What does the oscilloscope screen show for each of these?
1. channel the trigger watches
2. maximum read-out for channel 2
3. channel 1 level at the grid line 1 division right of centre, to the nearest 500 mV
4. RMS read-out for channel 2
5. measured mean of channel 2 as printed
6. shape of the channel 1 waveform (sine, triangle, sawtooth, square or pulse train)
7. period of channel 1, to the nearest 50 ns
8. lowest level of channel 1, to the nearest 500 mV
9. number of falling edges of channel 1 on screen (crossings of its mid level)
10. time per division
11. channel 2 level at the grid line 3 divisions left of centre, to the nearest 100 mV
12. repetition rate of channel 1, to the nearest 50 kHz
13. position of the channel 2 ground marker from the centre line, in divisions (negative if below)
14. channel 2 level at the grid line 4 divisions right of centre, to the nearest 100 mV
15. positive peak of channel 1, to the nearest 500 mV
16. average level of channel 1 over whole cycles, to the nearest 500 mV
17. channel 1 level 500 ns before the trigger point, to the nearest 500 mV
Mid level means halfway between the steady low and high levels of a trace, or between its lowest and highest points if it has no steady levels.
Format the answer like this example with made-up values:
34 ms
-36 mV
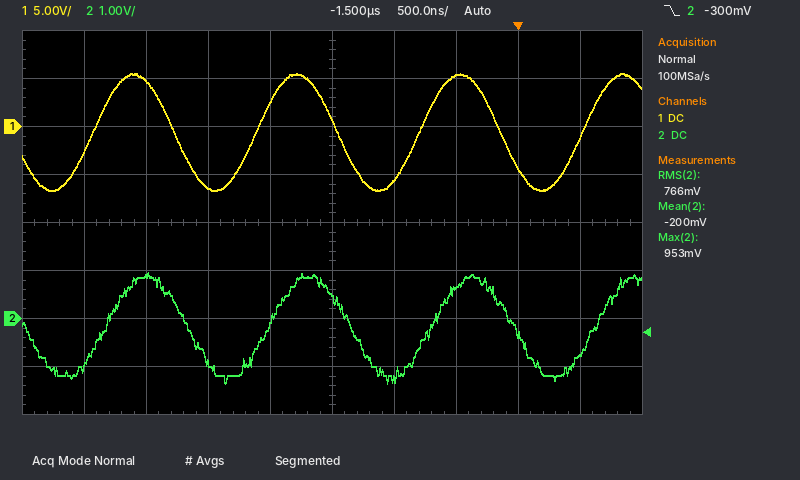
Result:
channel 2
953 mV
-5.5 V
766 mV
-200 mV
sine
1.30 µs
-6.5 V
3
500 ns
900 mV
750 kHz
-2.0 div
-700 mV
5.5 V
-500 mV
5.5 V
